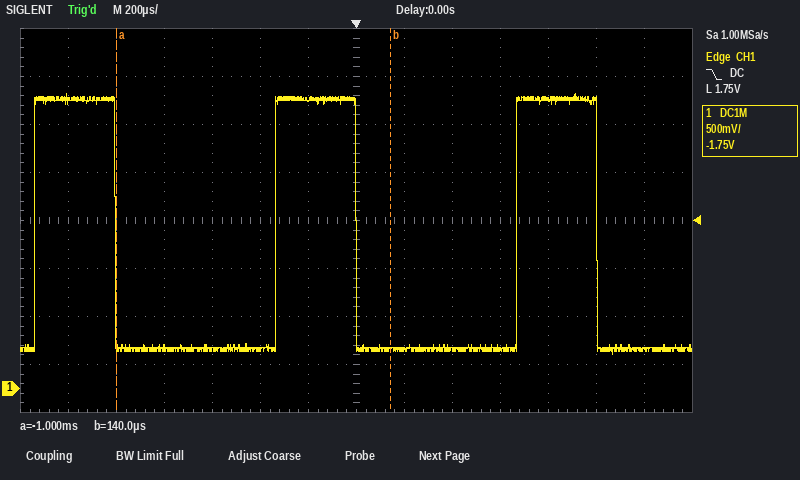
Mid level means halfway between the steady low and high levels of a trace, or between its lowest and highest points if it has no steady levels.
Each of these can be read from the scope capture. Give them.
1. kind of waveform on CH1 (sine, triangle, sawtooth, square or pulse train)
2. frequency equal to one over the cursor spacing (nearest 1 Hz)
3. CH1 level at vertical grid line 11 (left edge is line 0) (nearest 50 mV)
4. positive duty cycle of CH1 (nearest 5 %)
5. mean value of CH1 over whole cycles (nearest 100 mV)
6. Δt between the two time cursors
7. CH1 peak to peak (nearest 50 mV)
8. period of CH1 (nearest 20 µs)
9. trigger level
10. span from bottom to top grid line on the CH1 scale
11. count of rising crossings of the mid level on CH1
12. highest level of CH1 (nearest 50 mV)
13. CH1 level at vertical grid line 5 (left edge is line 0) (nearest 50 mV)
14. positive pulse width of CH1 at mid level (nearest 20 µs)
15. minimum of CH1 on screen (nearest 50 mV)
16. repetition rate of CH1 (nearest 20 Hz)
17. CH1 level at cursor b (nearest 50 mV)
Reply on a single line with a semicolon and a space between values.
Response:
pulse train; 877 Hz; 3.00 V; 35 %; 1.3 V; 1.14 ms; 2.70 V; 1.00 ms; 1.75 V; 4 V; 3; 3.05 V; 400 mV; 340 µs; 350 mV; 1.00 kHz; 400 mV
